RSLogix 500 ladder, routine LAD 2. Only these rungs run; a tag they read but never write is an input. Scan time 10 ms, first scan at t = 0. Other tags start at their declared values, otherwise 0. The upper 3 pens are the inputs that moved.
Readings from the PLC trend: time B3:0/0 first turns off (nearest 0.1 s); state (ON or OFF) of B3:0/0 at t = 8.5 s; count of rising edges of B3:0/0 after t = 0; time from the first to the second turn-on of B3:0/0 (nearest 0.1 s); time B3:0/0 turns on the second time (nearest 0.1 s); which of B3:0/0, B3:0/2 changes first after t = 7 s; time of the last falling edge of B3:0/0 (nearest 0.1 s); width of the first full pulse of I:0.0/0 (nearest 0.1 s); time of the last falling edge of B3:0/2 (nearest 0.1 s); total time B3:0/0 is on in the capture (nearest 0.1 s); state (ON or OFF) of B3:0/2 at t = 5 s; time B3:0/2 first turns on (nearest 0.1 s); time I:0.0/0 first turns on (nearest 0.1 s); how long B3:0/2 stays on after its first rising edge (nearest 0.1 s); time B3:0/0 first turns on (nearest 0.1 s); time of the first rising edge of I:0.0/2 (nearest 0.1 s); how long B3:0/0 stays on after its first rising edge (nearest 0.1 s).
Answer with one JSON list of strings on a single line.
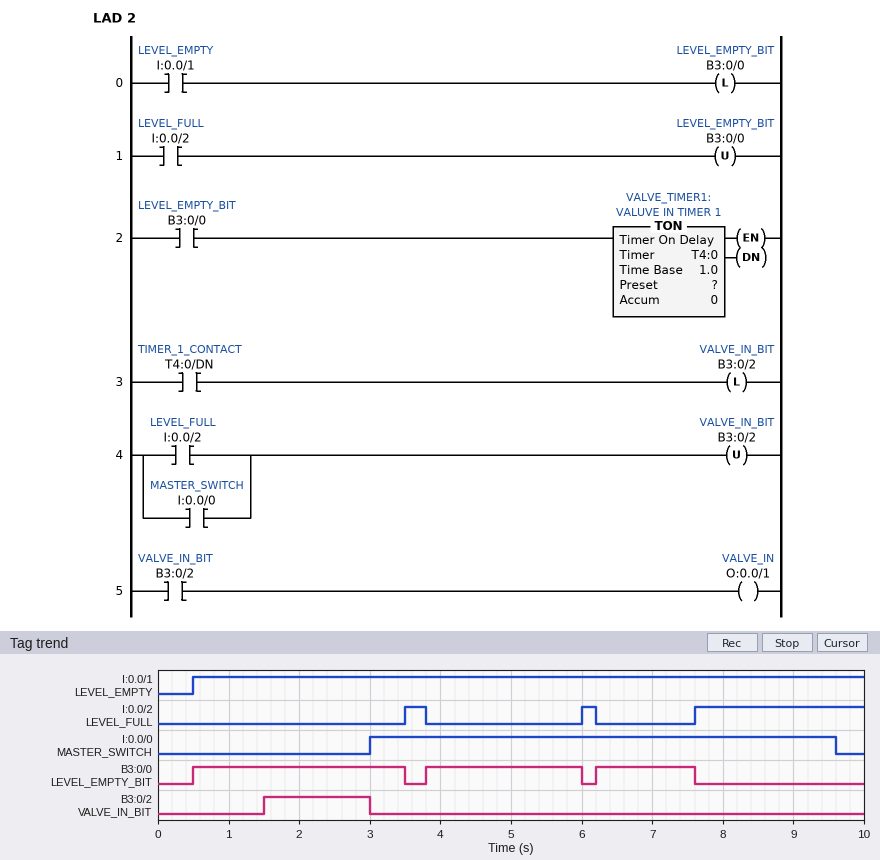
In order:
["3.5 s", "OFF", "3", "3.3 s", "3.8 s", "B3:0/0", "7.6 s", "6.6 s", "3.0 s", "6.6 s", "OFF", "1.5 s", "3.0 s", "1.5 s", "0.5 s", "3.5 s", "3.0 s"]
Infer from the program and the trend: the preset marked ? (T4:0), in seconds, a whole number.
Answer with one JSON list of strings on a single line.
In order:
["1 s"]
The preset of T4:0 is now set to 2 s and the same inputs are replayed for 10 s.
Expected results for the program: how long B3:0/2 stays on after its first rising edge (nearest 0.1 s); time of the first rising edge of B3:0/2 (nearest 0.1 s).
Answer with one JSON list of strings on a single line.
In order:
["0.5 s", "2.5 s"]
